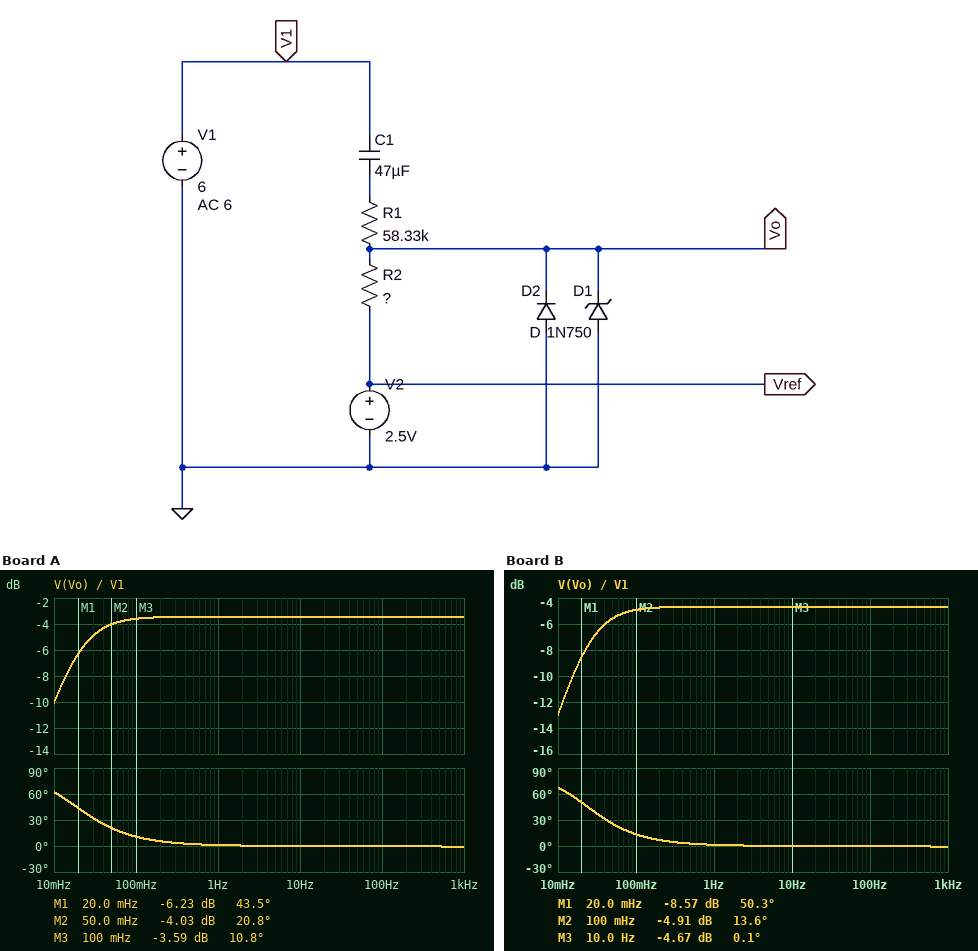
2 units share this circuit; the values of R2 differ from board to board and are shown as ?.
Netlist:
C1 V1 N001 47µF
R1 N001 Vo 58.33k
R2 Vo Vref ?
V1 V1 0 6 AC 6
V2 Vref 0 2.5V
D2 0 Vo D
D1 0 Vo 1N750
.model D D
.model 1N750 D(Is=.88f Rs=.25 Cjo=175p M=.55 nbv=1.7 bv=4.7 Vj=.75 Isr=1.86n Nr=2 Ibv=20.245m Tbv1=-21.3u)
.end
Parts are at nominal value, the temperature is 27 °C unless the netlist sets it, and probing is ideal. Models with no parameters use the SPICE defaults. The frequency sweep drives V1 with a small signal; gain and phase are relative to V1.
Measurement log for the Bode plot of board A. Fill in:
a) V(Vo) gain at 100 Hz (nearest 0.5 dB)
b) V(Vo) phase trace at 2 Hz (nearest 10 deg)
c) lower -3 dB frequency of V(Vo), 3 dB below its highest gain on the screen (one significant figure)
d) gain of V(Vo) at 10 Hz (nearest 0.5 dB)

-3.5 dB
0 deg
20 mHz
-3.5 dB
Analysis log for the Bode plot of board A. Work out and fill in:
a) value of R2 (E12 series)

120 kΩ
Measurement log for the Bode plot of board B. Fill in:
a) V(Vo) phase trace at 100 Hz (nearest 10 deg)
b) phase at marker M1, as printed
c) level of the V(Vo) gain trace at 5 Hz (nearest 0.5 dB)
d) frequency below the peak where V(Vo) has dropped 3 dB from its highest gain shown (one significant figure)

0 deg
50.3 deg
-4.5 dB
20 mHz
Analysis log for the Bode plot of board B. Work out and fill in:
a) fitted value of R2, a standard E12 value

82 kΩ
